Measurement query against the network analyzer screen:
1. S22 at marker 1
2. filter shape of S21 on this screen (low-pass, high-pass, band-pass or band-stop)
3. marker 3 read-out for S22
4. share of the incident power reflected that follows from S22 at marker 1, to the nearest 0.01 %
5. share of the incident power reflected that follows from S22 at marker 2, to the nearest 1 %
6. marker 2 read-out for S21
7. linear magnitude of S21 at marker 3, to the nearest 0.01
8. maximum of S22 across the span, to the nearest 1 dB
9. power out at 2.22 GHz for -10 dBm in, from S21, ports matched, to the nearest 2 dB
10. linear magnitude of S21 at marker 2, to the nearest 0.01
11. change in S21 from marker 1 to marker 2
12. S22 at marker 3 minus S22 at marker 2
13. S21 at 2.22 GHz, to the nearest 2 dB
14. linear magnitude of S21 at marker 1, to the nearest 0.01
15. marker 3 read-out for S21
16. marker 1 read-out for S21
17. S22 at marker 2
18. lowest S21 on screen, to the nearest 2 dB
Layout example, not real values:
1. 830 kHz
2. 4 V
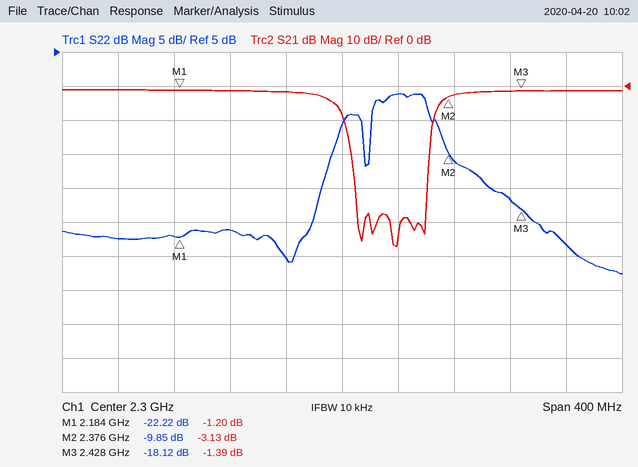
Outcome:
1. -22.22 dB
2. band-stop
3. -18.12 dB
4. 0.60 %
5. 10 %
6. -3.13 dB
7. 0.85
8. -1 dB
9. -12 dBm
10. 0.70
11. -1.93 dB
12. -8.27 dB
13. -2 dB
14. 0.87
15. -1.39 dB
16. -1.20 dB
17. -9.85 dB
18. -48 dB
